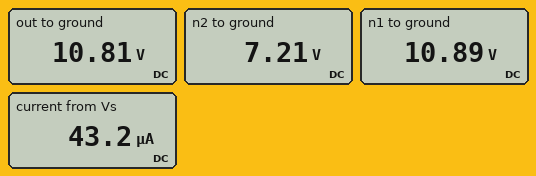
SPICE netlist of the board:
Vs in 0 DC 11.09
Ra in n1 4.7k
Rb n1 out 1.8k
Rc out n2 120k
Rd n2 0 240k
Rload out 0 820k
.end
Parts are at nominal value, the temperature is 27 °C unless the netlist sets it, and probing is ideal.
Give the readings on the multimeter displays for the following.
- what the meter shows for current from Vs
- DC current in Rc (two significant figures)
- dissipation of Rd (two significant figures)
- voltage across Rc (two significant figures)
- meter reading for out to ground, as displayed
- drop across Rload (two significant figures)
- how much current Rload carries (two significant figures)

43.2 µA
30 µA
220 µW
3.6 V
10.81 V
11 V
13 µA
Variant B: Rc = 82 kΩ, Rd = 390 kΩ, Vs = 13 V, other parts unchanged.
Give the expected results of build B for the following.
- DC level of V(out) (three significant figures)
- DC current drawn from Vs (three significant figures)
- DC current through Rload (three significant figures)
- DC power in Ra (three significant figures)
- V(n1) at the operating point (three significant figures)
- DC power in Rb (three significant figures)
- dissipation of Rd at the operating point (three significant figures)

12.7 V
42.5 µA
15.5 µA
8.48 µW
12.8 V
3.25 µW
283 µW
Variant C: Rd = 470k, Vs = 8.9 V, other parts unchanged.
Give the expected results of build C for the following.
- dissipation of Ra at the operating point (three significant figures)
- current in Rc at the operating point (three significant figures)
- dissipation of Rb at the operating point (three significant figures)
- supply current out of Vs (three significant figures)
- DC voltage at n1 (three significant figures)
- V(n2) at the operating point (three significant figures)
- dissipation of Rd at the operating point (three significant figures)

3.05 µW
14.8 µA
1.17 µW
25.5 µA
8.78 V
6.96 V
103 µW
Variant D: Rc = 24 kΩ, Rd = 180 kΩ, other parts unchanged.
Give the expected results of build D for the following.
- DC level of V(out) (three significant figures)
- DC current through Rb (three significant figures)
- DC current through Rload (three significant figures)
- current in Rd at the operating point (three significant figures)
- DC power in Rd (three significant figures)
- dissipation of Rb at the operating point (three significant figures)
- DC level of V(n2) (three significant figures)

10.7 V
65.3 µA
13.0 µA
52.3 µA
492 µW
7.67 µW
9.41 V
